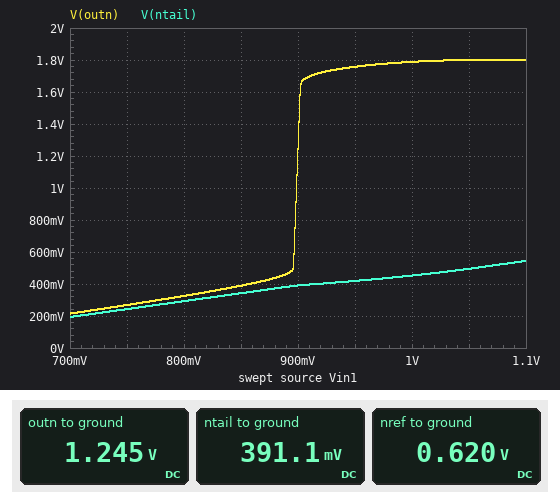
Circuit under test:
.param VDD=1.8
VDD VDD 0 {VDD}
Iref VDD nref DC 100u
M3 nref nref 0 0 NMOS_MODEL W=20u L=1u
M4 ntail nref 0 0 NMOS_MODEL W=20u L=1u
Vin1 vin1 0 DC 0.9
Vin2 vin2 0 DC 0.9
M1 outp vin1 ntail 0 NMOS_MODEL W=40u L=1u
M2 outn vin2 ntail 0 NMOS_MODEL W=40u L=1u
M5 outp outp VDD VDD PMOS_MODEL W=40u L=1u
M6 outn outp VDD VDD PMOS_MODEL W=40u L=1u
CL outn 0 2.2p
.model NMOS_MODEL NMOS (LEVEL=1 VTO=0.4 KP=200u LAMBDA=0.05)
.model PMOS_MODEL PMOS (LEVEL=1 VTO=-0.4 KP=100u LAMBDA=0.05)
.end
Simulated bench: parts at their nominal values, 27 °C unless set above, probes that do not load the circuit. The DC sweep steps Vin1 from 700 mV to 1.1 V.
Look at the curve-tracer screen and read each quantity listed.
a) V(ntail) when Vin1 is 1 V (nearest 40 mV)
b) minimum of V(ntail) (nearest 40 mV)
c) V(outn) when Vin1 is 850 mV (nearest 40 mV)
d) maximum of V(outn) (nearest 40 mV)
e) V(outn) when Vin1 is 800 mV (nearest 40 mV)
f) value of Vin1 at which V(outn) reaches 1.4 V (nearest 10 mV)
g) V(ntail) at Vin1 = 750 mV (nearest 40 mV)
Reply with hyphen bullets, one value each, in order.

- 440 mV
- 200 mV
- 400 mV
- 1.80 V
- 320 mV
- 900 mV
- 240 mV
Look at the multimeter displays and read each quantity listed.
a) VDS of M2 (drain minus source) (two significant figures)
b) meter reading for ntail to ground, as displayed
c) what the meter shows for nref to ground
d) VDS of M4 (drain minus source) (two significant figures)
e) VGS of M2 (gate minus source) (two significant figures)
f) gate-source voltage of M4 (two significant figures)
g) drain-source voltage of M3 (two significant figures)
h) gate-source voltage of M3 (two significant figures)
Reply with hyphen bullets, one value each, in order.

- 850 mV
- 391.1 mV
- 0.620 V
- 390 mV
- 510 mV
- 620 mV
- 620 mV
- 620 mV
